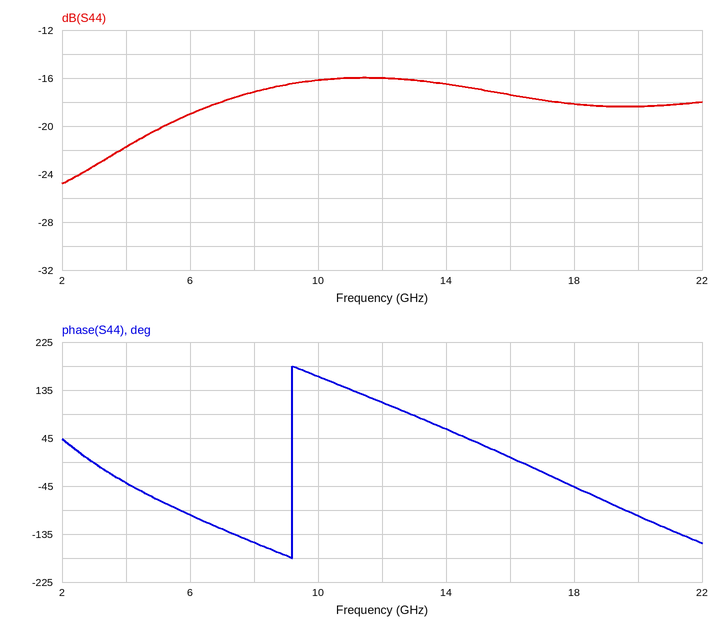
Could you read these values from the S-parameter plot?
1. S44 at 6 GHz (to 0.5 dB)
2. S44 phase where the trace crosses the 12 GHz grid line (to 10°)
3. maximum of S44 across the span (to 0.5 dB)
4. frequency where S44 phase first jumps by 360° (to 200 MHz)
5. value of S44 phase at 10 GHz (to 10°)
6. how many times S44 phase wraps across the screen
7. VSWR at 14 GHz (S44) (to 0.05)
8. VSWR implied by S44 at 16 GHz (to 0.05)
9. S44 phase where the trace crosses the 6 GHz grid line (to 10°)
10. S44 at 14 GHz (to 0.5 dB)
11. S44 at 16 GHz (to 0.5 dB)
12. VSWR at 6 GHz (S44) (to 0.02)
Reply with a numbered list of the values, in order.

1. -19.0 dB
2. 110°
3. -16.0 dB
4. 9.2 GHz
5. 160°
6. 1
7. 1.35
8. 1.30
9. -100°
10. -16.5 dB
11. -17.5 dB
12. 1.26
